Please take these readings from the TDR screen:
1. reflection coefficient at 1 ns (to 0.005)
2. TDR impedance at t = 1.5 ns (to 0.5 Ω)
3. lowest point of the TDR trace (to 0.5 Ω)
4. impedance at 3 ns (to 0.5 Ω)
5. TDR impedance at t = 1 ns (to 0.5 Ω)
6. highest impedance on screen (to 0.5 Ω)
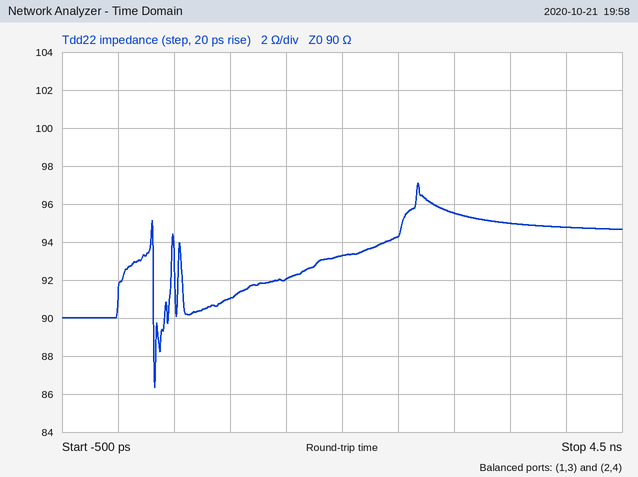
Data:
+0.005
92.0 Ω
86.5 Ω
95.5 Ω
91.0 Ω
97.0 Ω
